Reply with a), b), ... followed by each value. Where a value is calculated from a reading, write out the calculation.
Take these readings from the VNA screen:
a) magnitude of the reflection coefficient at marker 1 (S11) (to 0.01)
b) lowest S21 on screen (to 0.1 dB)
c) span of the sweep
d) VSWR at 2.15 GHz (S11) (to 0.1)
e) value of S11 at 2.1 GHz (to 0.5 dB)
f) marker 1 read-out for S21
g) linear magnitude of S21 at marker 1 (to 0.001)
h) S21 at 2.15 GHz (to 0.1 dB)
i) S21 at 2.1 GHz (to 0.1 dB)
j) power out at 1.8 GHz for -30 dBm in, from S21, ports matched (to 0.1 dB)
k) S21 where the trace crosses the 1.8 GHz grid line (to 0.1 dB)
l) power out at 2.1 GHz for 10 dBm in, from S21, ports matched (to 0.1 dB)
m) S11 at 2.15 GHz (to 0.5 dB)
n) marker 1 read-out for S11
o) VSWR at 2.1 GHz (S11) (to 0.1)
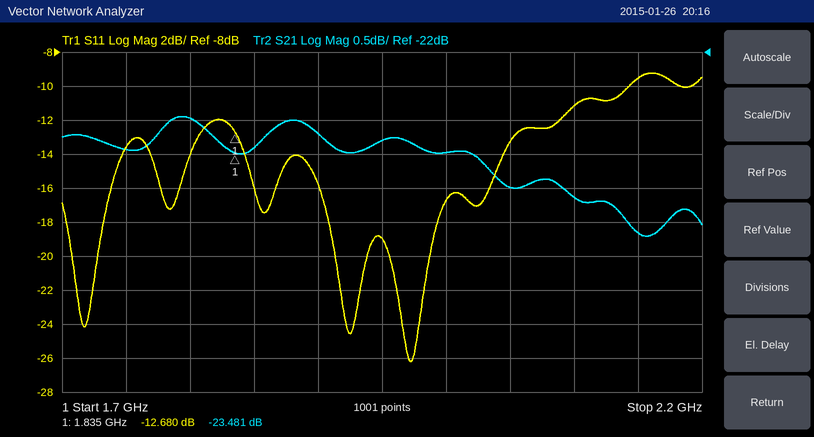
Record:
a) 10^(-12.68/20) ≈ 0.23
b) -24.7 dB
c) 500 MHz
d) |Γ| = 10^(-9.5/20) = 0.3350; VSWR = (1 + 0.3350)/(1 − 0.3350) ≈ 2.0
e) -11.0 dB
f) -23.481 dB
g) 10^(-23.481/20) ≈ 0.067
h) -24.7 dB
i) -24.1 dB
j) -30 dBm + (-23.0 dB) = -53.0 dBm
k) -23.0 dB
l) 10 dBm + (-24.1 dB) = -14.1 dBm
m) -9.5 dB
n) -12.680 dB
o) |Γ| = 10^(-11/20) = 0.2818; VSWR = (1 + 0.2818)/(1 − 0.2818) ≈ 1.8
